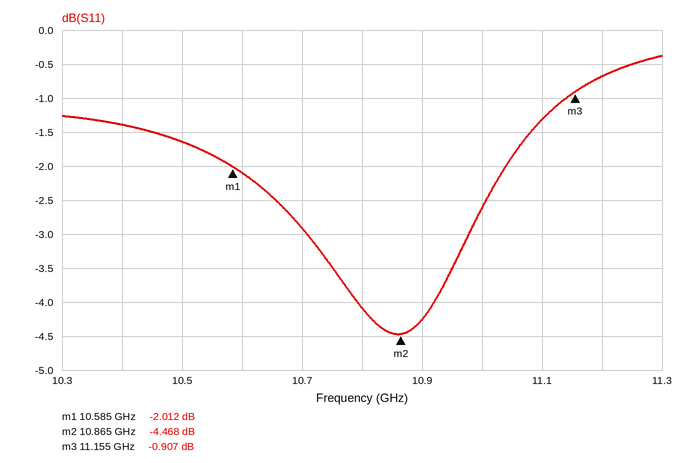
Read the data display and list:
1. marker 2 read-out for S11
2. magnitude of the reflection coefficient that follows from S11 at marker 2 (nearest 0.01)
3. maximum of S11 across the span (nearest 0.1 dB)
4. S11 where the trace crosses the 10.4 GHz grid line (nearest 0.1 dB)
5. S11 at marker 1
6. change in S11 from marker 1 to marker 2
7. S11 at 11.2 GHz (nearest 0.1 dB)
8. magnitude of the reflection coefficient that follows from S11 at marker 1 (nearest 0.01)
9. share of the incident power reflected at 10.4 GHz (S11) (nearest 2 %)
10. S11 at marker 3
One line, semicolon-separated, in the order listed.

-4.468 dB; 0.60; -0.4 dB; -1.4 dB; -2.012 dB; -2.456 dB; -0.7 dB; 0.79; 72 %; -0.907 dB
